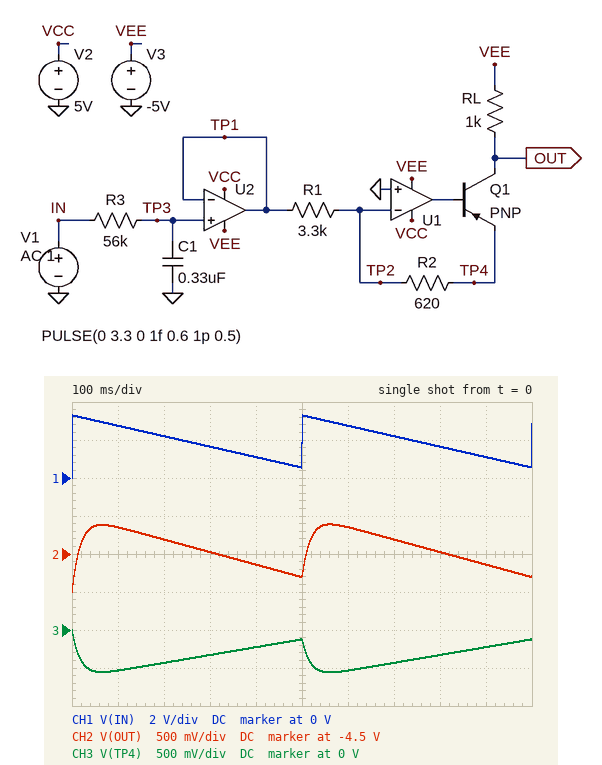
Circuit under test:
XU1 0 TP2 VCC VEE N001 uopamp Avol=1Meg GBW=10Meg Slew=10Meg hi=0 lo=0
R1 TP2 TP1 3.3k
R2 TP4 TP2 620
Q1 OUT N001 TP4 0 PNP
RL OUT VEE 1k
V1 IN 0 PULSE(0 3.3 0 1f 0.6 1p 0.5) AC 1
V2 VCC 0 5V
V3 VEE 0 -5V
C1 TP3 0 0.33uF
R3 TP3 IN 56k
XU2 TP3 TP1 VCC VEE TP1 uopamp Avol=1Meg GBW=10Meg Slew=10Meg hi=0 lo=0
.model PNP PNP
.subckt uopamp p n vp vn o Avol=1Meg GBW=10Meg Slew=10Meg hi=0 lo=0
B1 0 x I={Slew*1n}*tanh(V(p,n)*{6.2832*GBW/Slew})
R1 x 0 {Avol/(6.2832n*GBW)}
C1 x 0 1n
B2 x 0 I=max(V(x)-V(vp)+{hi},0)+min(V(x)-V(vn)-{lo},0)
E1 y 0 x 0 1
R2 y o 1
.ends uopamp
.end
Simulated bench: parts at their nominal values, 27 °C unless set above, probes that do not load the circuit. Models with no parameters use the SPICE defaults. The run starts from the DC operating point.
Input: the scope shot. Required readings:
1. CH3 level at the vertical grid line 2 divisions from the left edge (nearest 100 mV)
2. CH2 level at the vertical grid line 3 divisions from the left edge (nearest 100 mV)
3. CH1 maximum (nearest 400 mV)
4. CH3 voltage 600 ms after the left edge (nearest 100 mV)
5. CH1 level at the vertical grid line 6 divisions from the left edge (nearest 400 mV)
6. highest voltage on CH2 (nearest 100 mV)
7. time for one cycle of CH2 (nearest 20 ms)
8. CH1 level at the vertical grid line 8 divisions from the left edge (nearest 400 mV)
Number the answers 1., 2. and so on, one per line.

1. -400 mV
2. -4.5 V
3. 3.2 V
4. -500 mV
5. 2.8 V
6. -4.1 V
7. 500 ms
8. 1.6 V
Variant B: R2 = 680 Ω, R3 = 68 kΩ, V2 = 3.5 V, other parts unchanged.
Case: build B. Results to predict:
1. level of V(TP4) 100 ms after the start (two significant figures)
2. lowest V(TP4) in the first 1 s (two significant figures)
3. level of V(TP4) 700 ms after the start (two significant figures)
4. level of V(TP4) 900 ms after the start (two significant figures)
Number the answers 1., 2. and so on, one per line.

1. -580 mV
2. -600 mV
3. -480 mV
4. -250 mV
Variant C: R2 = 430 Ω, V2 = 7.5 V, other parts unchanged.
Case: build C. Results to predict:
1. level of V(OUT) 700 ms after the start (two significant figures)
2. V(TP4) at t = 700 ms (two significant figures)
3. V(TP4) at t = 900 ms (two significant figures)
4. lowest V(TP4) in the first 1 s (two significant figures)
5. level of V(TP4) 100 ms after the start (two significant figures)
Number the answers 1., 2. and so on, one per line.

1. -4.3 V
2. -300 mV
3. -160 mV
4. -390 mV
5. -370 mV
